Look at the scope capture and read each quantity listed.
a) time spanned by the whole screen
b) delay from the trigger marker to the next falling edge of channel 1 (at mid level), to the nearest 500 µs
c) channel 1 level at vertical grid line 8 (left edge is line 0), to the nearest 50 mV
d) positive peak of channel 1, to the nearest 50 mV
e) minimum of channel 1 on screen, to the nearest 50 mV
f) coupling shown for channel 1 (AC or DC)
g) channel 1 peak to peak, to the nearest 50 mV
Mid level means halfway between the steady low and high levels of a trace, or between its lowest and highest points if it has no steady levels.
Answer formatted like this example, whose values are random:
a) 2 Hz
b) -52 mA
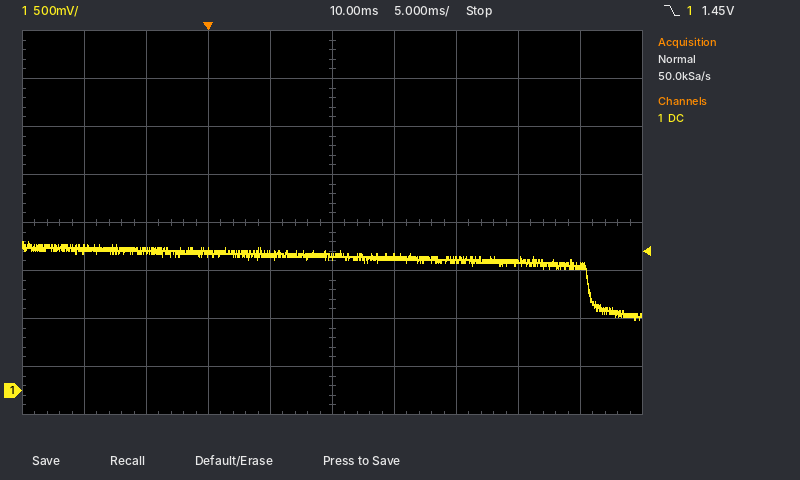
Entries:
a) 50 ms
b) 30.5 ms
c) 1.35 V
d) 1.55 V
e) 750 mV
f) DC
g) 800 mV
